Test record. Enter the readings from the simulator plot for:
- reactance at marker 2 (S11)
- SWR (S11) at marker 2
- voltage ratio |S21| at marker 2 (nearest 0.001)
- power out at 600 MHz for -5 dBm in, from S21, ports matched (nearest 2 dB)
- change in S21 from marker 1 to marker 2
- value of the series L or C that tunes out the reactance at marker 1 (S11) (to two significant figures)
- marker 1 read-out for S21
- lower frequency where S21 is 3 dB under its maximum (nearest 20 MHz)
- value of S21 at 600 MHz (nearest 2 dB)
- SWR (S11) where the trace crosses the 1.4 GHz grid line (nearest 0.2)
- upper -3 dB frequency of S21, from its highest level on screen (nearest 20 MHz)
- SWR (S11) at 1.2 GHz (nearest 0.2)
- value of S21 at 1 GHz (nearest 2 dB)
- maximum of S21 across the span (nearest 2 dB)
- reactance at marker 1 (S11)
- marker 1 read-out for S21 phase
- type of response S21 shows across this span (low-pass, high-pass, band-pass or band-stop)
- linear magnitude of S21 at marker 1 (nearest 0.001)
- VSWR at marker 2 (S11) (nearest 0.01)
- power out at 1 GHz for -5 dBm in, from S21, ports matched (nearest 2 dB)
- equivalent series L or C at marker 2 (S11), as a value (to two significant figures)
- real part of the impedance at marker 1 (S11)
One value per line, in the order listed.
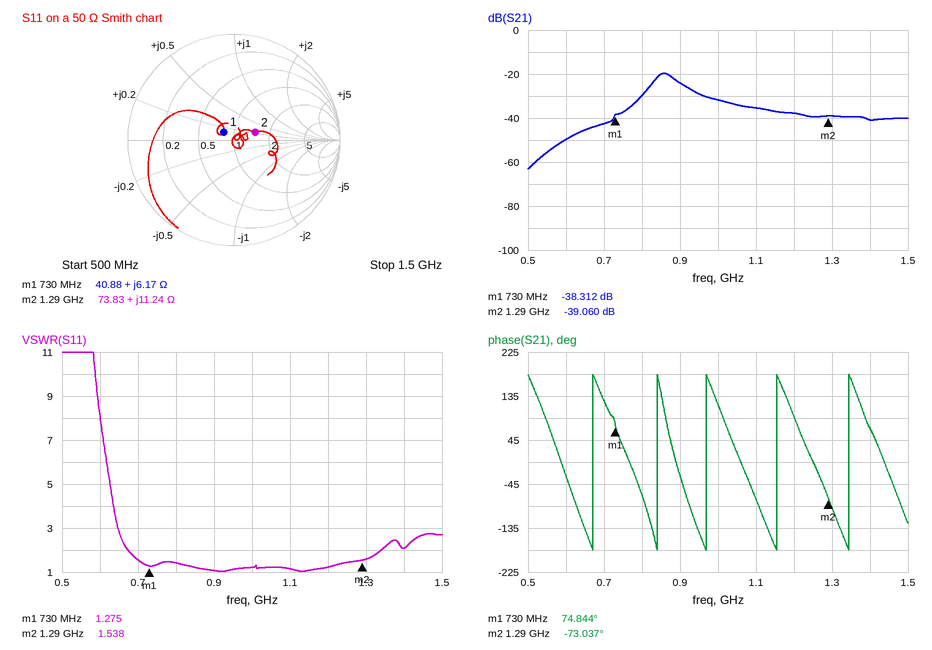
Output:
+11.24 Ω
1.538
0.011
-54 dBm
-0.748 dB
35 pF
-38.312 dB
840 MHz
-50 dB
2.0
880 MHz
1.2
-32 dB
-20 dB
+6.17 Ω
74.844°
band-pass
0.012
1.54
-36 dBm
1.4 nH
40.88 Ω
